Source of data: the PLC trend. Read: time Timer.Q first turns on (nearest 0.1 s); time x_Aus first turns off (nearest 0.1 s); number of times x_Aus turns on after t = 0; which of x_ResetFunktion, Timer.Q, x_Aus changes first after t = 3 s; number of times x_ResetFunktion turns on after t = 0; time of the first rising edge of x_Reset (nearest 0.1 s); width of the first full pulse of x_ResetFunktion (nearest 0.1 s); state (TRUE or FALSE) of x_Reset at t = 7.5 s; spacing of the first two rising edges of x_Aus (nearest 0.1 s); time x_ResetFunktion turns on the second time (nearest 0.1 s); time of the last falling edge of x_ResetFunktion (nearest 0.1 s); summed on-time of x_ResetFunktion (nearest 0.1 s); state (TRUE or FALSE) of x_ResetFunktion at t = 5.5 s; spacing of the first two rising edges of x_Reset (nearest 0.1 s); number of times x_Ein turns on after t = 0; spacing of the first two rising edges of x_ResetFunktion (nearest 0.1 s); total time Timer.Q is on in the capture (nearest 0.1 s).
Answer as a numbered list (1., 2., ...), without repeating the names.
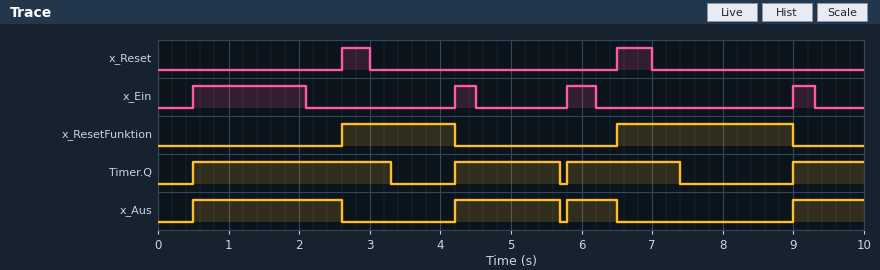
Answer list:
1. 0.5 s
2. 2.6 s
3. 4
4. Timer.Q
5. 2
6. 2.6 s
7. 1.6 s
8. FALSE
9. 3.7 s
10. 6.5 s
11. 9.0 s
12. 4.1 s
13. FALSE
14. 3.9 s
15. 4
16. 3.9 s
17. 6.9 s
